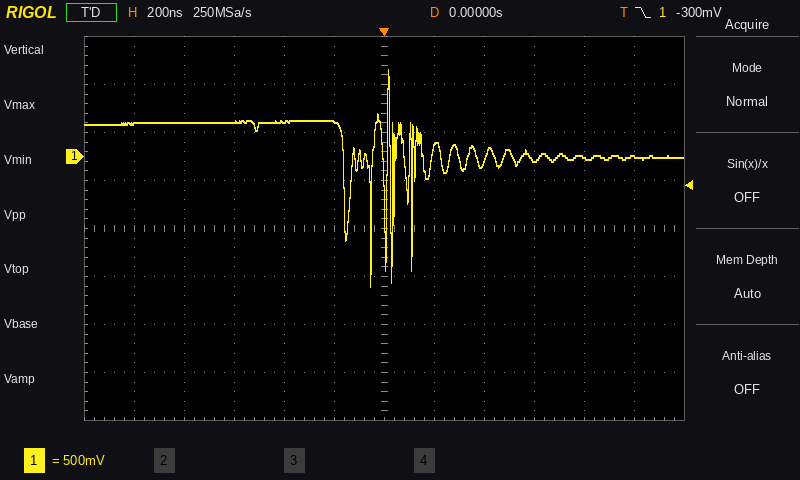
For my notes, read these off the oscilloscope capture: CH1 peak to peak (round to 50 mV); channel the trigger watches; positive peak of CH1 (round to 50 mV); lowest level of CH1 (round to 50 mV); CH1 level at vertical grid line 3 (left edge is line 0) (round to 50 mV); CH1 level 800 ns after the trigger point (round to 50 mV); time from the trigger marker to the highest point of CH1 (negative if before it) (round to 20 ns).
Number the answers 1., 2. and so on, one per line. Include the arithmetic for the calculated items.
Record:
1. 900 mV − (-1.35 V) = 2.25 V
2. CH1
3. 900 mV
4. -1.35 V
5. 350 mV
6. 0 mV
7. +20 ns
